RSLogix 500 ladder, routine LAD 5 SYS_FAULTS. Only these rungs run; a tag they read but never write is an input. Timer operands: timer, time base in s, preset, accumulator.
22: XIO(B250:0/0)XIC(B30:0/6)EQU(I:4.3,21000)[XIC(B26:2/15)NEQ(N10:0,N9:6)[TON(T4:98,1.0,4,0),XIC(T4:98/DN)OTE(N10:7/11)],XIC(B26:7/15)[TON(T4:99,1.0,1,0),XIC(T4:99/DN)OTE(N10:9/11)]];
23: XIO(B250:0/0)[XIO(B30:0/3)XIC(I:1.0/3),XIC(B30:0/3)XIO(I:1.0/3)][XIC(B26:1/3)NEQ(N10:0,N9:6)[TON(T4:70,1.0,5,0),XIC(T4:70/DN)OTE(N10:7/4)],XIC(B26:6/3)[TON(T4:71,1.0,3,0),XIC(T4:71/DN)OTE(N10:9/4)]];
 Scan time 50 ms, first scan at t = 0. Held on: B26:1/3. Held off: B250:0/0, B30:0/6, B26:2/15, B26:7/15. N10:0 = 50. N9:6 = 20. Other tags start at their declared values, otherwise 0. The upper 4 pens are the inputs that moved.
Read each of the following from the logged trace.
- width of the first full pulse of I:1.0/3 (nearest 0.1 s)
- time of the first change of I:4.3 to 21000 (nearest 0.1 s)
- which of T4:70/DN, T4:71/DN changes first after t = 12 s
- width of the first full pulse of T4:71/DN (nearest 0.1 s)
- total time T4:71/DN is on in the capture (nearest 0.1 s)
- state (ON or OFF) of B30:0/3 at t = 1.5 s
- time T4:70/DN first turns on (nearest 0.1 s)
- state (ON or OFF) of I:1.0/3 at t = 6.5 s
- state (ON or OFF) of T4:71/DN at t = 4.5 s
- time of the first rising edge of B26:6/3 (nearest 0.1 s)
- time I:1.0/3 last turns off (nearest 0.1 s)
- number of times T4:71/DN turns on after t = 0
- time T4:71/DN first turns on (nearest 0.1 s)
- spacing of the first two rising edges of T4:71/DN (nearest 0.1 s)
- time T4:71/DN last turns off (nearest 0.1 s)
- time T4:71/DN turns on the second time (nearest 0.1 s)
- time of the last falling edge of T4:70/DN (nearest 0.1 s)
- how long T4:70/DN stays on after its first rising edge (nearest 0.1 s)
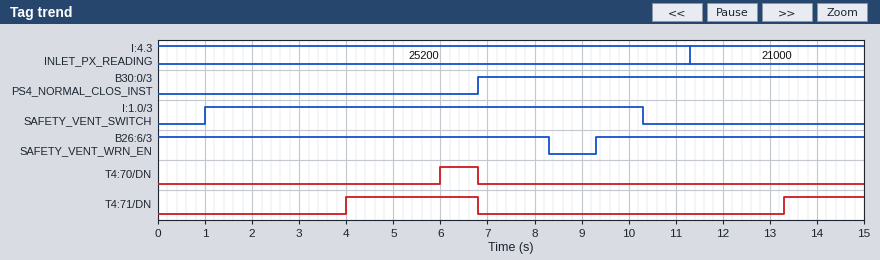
9.3 s
11.3 s
T4:71/DN
2.8 s
4.5 s
OFF
6.0 s
ON
ON
9.3 s
10.3 s
2
4.0 s
9.3 s
6.8 s
13.3 s
6.8 s
0.8 s
